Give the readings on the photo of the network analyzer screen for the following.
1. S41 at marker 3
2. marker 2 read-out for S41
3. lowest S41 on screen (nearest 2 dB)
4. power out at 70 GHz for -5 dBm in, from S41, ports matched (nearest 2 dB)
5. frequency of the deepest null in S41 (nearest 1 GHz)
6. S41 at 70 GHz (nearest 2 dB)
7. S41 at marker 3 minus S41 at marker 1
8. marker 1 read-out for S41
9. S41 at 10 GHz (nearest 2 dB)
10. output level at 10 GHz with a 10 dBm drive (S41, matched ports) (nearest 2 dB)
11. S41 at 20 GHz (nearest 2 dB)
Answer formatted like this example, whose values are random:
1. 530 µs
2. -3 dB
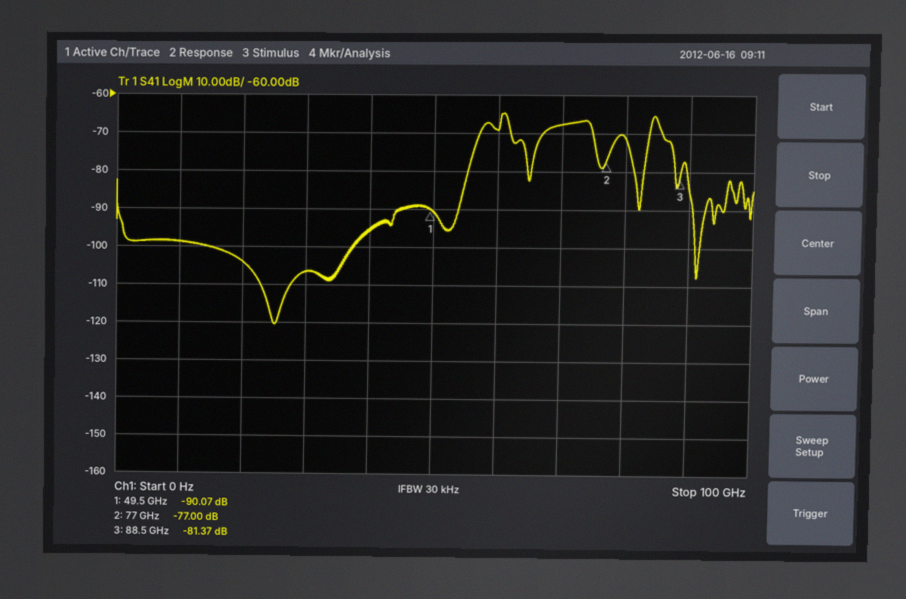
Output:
1. -81.37 dB
2. -77.00 dB
3. -120 dB
4. -72 dBm
5. 25 GHz
6. -68 dB
7. 8.70 dB
8. -90.07 dB
9. -98 dB
10. -88 dBm
11. -104 dB
